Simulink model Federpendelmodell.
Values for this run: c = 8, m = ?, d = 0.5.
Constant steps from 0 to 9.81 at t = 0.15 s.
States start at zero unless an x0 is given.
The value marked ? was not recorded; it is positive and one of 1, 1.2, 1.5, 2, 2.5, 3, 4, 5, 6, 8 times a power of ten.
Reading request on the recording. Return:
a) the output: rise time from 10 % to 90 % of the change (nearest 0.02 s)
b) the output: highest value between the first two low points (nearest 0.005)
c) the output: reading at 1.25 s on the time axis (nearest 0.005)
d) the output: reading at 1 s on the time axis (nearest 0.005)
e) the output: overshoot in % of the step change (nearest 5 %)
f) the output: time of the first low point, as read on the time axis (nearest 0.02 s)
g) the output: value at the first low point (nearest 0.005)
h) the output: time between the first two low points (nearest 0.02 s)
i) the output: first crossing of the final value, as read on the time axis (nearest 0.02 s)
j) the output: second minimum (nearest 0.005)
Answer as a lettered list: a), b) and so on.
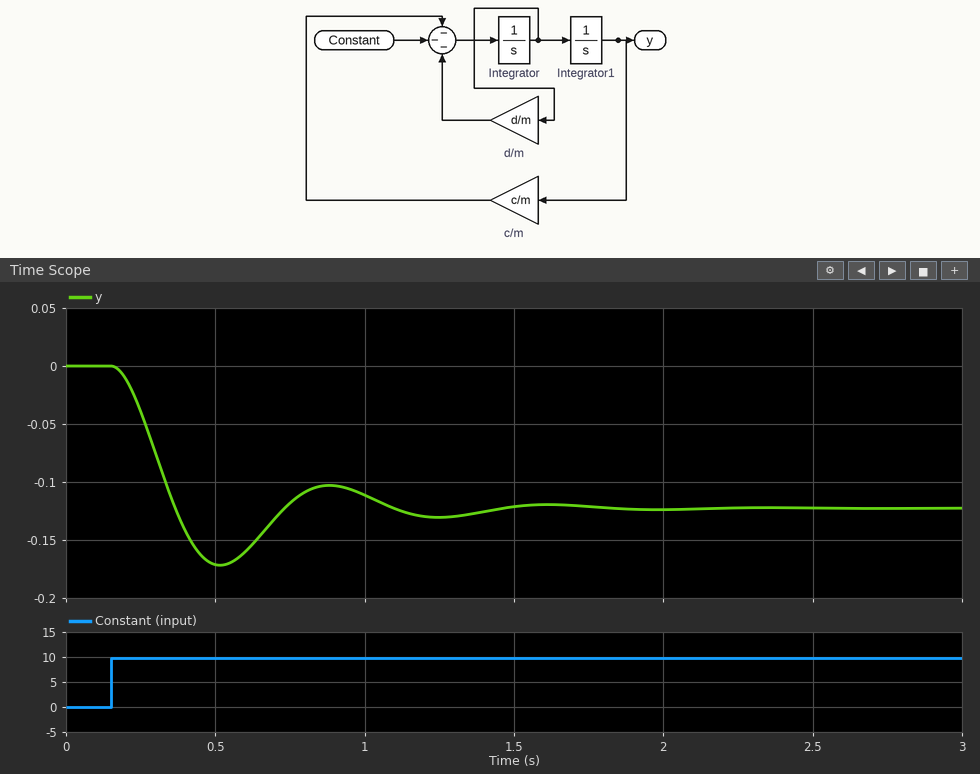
a) 0.14 s
b) -0.105
c) -0.130
d) -0.110
e) 40 %
f) 0.52 s
g) -0.170
h) 0.74 s
i) 0.36 s
j) -0.130
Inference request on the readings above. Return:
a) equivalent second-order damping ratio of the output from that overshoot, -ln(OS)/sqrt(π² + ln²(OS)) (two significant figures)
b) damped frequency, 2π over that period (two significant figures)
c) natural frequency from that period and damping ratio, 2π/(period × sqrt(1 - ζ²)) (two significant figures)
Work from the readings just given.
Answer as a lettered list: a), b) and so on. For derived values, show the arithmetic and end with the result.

a) ln(0.4) = -0.916; 0.916 / sqrt(9.870 + 0.840) = 0.28
b) 2π / 0.74 = 8.5 rad/s
c) 2π / (0.74 × sqrt(1 - 0.28²)) = 8.8 rad/s
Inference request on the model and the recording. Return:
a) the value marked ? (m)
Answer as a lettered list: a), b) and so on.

a) 0.1
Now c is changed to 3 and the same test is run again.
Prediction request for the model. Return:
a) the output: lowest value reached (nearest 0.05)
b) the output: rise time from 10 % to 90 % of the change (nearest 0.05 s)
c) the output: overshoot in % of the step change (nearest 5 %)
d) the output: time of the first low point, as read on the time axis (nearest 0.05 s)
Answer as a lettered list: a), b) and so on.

a) -0.40
b) 0.30 s
c) 20 %
d) 0.80 s
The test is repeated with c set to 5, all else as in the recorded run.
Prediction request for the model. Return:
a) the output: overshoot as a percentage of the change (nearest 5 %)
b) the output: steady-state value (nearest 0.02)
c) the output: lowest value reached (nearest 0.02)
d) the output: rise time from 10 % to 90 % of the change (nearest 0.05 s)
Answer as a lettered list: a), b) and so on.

a) 30 %
b) -0.20
c) -0.26
d) 0.20 s
